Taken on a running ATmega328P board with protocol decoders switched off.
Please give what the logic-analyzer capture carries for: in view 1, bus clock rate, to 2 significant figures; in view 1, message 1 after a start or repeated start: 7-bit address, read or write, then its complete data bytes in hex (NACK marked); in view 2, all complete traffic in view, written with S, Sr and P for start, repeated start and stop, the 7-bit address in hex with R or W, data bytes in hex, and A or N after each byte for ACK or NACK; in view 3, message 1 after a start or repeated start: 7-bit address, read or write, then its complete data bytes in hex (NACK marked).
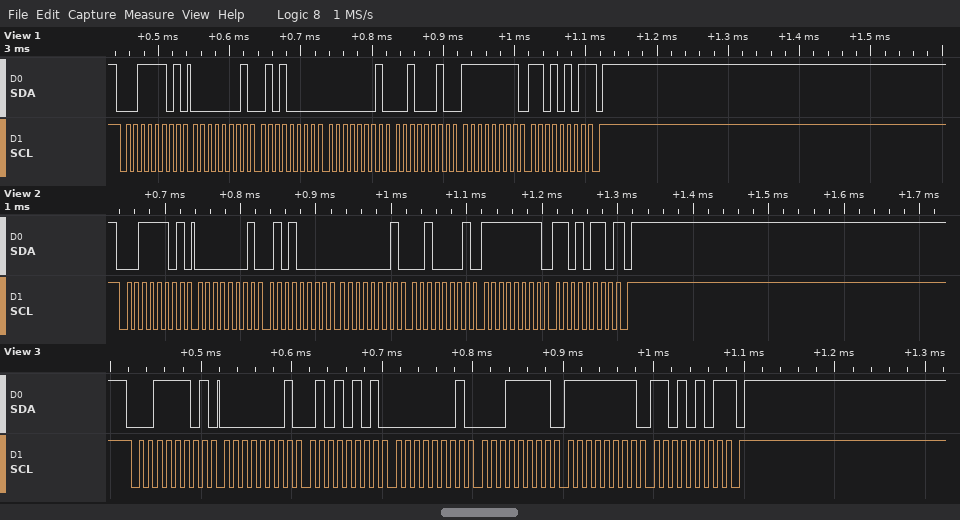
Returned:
100 kHz
0x1E read: 01 50 01 22 FF D5 NACK
S 1ER A 01 A 50 A 01 A 21 A FF A D6 N P
0x1E read: 01 55 01 1F FF D5 NACK
